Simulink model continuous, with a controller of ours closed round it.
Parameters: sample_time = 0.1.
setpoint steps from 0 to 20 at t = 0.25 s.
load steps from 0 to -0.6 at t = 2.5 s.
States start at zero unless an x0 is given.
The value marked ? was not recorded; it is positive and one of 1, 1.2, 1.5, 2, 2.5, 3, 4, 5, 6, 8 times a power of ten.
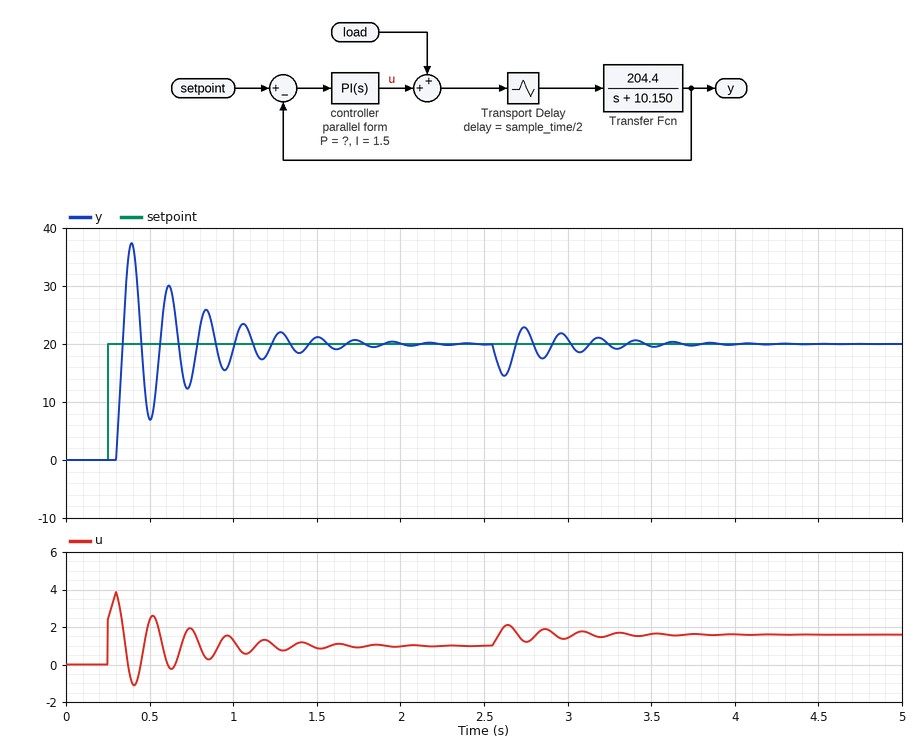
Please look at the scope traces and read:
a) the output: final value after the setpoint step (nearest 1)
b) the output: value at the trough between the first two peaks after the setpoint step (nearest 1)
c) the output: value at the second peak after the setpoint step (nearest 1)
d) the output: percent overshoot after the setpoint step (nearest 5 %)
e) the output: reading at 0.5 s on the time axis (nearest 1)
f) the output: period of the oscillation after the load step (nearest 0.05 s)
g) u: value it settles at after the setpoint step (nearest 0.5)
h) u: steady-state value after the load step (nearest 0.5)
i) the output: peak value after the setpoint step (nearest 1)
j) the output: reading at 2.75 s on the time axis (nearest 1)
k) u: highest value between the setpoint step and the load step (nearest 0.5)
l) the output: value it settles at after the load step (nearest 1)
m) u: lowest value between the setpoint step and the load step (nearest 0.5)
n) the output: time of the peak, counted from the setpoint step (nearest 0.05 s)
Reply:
20
7
30
85 %
7
0.25 s
1.0
1.5
37
23
4.0
20
-1.0
0.15 s
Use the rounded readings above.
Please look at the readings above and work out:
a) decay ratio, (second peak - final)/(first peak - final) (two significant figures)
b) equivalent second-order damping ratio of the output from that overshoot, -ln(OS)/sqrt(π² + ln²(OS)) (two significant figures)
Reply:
0.59
0.052
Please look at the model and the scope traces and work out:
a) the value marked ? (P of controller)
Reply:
0.12
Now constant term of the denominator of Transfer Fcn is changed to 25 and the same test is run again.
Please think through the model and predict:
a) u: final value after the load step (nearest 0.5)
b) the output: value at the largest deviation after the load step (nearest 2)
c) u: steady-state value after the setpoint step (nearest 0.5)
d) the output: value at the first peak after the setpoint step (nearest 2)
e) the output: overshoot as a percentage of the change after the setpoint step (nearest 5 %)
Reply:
3.0
16
2.5
24
20 %
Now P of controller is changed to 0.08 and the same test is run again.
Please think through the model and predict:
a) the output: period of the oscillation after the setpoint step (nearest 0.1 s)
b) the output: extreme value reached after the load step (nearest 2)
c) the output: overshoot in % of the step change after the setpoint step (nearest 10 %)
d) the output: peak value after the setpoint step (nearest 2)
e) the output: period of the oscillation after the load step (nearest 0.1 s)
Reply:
0.3 s
14
80 %
36
0.3 s
